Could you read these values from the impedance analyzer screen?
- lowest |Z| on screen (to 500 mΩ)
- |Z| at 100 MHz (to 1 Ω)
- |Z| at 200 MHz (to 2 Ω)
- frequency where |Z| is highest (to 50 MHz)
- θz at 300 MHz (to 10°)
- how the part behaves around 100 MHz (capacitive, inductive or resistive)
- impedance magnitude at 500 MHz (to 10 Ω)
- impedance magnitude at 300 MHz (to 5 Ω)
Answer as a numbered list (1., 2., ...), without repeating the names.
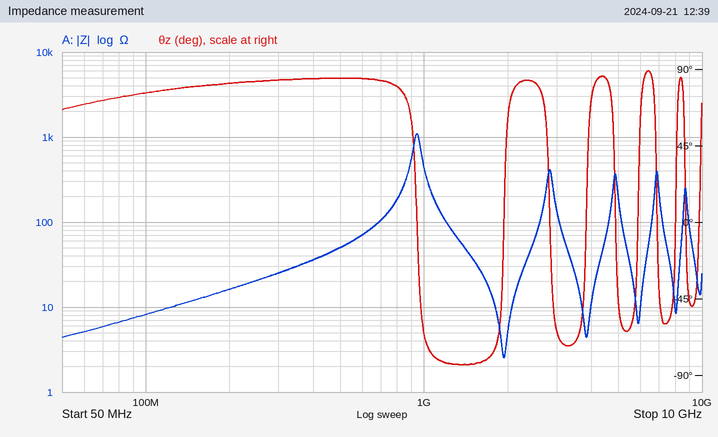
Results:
1. 2.5 Ω
2. 8 Ω
3. 16 Ω
4. 950 MHz
5. 80°
6. inductive
7. 50 Ω
8. 25 Ω
